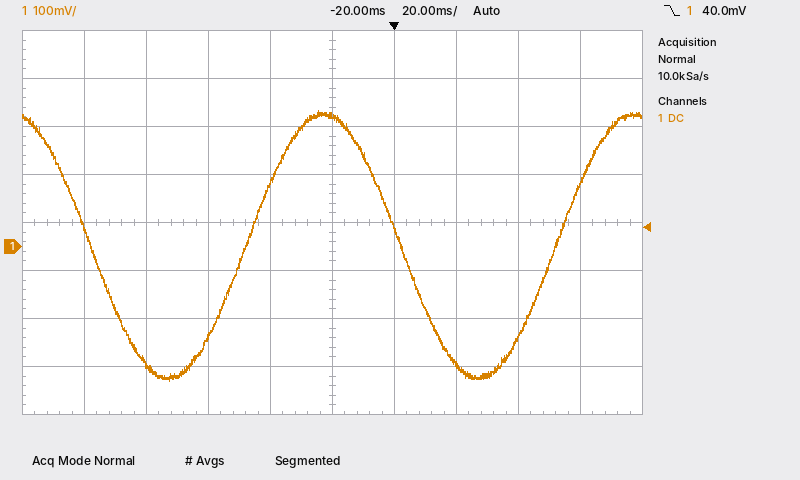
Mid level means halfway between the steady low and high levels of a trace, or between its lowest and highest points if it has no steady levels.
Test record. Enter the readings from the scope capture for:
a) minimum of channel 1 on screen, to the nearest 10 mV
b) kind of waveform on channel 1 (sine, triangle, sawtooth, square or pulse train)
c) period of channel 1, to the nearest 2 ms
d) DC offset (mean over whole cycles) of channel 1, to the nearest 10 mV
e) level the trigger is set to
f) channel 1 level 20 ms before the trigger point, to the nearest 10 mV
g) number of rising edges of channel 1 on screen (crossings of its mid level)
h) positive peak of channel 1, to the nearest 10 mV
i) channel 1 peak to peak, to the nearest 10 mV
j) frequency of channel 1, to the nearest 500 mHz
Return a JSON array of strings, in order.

["-280 mV", "sine", "100 ms", "0 mV", "40.0 mV", "270 mV", "2", "280 mV", "560 mV", "10.0 Hz"]
